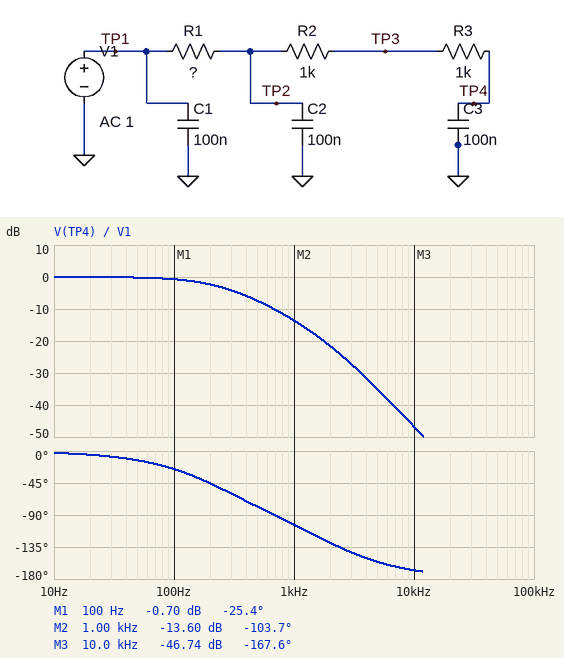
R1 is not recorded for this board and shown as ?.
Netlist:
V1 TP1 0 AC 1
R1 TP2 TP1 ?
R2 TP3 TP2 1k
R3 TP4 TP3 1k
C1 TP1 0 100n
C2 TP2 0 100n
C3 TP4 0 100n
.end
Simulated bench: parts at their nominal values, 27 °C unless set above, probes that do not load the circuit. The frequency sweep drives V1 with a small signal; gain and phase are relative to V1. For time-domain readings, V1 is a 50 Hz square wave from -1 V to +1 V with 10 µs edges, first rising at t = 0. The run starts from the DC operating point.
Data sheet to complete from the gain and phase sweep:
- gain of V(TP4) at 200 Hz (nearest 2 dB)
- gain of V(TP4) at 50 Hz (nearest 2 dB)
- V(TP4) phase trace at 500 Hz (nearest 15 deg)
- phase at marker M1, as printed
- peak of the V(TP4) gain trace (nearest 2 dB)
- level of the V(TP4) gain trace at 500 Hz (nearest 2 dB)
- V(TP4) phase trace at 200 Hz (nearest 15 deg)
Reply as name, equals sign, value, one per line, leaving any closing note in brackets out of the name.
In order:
gain of V(TP4) at 200 Hz = -2 dB
gain of V(TP4) at 50 Hz = 0 dB
V(TP4) phase trace at 500 Hz = -75 deg
phase at marker M1, as printed = -25.4 deg
peak of the V(TP4) gain trace = 0 dB
level of the V(TP4) gain trace at 500 Hz = -8 dB
V(TP4) phase trace at 200 Hz = -45 deg
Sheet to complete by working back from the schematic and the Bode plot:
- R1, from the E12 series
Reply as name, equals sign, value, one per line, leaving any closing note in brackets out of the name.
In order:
R1, from the E12 series = 2.7 kΩ
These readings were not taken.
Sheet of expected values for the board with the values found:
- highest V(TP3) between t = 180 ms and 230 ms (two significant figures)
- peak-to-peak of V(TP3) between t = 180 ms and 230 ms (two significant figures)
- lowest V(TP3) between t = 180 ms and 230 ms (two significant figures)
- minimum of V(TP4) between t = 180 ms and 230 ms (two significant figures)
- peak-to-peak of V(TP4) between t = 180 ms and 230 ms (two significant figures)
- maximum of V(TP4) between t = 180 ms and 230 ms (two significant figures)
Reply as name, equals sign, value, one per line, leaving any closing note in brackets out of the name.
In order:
highest V(TP3) between t = 180 ms and 230 ms = 1.0 V
peak-to-peak of V(TP3) between t = 180 ms and 230 ms = 2.0 V
lowest V(TP3) between t = 180 ms and 230 ms = -1.0 V
minimum of V(TP4) between t = 180 ms and 230 ms = -1.0 V
peak-to-peak of V(TP4) between t = 180 ms and 230 ms = 2.0 V
maximum of V(TP4) between t = 180 ms and 230 ms = 1.0 V
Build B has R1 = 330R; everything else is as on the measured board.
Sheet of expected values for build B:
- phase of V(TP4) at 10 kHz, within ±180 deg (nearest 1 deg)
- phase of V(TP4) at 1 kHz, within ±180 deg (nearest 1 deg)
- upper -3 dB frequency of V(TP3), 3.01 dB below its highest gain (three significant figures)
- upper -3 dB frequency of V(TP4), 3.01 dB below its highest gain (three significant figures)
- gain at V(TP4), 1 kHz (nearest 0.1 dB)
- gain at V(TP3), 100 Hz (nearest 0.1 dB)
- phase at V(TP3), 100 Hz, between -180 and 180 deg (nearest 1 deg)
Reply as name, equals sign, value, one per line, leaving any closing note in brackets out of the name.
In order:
phase of V(TP4) at 10 kHz, within ±180 deg = -146 deg
phase of V(TP4) at 1 kHz, within ±180 deg = -66 deg
upper -3 dB frequency of V(TP3), 3.01 dB below its highest gain = 809 Hz
upper -3 dB frequency of V(TP4), 3.01 dB below its highest gain = 659 Hz
gain at V(TP4), 1 kHz = -5.2 dB
gain at V(TP3), 100 Hz = -0.1 dB
phase at V(TP3), 100 Hz, between -180 and 180 deg = -6 deg
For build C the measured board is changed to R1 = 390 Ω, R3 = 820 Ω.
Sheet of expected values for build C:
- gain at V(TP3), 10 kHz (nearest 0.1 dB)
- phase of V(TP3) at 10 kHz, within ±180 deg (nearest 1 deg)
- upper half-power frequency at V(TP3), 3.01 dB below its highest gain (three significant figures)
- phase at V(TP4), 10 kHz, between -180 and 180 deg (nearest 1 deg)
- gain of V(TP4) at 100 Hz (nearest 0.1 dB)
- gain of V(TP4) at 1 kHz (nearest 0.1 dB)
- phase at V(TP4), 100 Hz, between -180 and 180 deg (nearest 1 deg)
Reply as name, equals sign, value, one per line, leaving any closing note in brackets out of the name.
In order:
gain at V(TP3), 10 kHz = -15.6 dB
phase of V(TP3) at 10 kHz, within ±180 deg = -70 deg
upper half-power frequency at V(TP3), 3.01 dB below its highest gain = 784 Hz
phase at V(TP4), 10 kHz, between -180 and 180 deg = -149 deg
gain of V(TP4) at 100 Hz = -0.1 dB
gain of V(TP4) at 1 kHz = -5.0 dB
phase at V(TP4), 100 Hz, between -180 and 180 deg = -9 deg
